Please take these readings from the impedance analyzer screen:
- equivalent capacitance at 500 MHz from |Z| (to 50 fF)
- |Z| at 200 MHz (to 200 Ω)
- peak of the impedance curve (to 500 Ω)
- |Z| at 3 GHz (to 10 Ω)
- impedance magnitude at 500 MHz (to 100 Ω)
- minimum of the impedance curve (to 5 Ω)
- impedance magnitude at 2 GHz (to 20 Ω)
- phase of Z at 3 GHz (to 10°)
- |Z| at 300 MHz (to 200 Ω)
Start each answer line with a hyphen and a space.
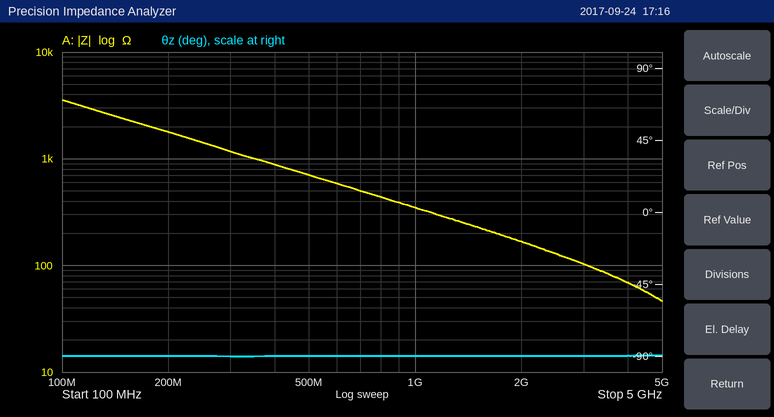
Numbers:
- 450 fF
- 1.8 kΩ
- 3.5 kΩ
- 100 Ω
- 700 Ω
- 45 Ω
- 160 Ω
- -90°
- 1.2 kΩ
